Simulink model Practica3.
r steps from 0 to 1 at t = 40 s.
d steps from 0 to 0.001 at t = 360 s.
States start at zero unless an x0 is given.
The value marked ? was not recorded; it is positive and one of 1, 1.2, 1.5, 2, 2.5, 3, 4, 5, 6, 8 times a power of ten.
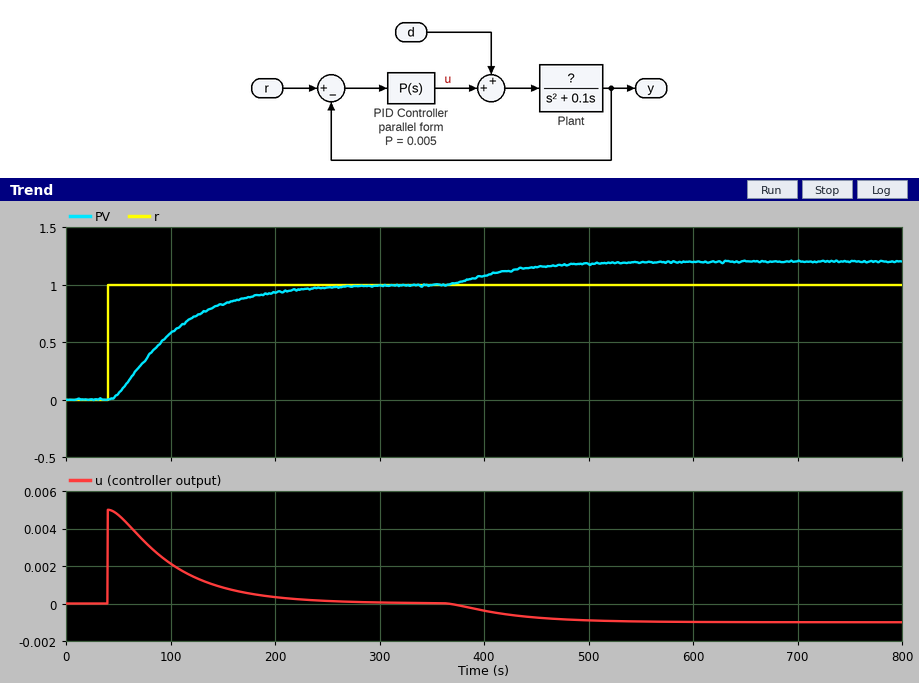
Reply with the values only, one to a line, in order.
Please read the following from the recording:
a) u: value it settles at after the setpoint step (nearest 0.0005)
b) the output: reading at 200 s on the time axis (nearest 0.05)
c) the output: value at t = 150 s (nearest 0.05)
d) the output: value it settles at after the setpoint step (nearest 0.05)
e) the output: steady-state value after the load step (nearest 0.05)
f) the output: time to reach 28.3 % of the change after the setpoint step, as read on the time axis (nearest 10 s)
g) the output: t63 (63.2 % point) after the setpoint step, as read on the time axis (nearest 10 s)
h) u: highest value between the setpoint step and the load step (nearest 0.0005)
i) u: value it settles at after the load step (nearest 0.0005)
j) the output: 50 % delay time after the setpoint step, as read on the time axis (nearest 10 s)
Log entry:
0.0000
0.95
0.85
1.00
1.20
70 s
110 s
0.0050
-0.0010
90 s
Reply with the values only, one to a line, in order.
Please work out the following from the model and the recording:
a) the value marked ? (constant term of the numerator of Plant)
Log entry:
0.3
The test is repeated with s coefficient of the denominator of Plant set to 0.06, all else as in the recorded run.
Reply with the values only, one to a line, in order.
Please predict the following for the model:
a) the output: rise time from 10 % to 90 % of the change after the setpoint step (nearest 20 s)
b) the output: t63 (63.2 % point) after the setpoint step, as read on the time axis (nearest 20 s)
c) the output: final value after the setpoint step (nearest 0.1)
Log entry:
60 s
80 s
1.0
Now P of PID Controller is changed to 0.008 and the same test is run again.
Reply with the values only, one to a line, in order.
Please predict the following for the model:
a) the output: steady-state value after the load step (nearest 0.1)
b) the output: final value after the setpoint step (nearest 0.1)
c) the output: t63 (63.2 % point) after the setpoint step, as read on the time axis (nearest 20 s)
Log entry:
1.1
1.0
80 s
